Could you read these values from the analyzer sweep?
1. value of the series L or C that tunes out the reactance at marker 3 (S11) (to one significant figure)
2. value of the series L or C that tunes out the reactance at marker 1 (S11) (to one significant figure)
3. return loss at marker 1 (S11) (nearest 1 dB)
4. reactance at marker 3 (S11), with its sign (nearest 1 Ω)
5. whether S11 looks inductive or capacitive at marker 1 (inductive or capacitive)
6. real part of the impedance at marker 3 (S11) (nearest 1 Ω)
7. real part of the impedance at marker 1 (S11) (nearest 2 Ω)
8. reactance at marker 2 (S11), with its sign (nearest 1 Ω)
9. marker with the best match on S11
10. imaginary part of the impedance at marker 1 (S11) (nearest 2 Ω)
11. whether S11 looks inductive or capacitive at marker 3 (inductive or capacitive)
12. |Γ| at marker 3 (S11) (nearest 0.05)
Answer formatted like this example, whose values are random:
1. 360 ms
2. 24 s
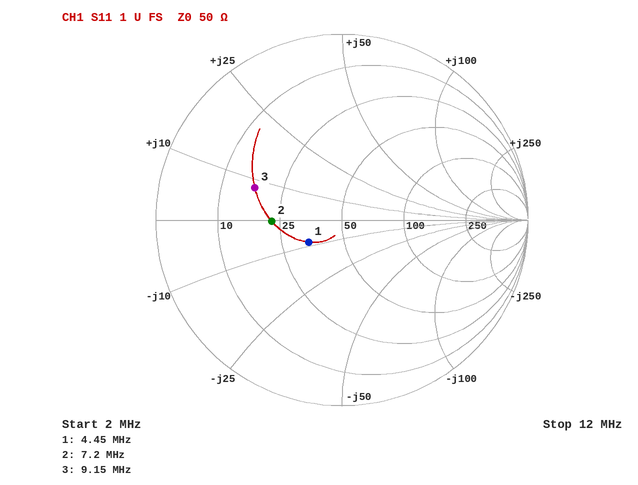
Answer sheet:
1. 2 nF
2. 300 nH
3. 13 dB
4. +8 Ω
5. capacitive
6. 17 Ω
7. 34 Ω
8. 0 Ω
9. marker 1
10. -8 Ω
11. inductive
12. 0.50
